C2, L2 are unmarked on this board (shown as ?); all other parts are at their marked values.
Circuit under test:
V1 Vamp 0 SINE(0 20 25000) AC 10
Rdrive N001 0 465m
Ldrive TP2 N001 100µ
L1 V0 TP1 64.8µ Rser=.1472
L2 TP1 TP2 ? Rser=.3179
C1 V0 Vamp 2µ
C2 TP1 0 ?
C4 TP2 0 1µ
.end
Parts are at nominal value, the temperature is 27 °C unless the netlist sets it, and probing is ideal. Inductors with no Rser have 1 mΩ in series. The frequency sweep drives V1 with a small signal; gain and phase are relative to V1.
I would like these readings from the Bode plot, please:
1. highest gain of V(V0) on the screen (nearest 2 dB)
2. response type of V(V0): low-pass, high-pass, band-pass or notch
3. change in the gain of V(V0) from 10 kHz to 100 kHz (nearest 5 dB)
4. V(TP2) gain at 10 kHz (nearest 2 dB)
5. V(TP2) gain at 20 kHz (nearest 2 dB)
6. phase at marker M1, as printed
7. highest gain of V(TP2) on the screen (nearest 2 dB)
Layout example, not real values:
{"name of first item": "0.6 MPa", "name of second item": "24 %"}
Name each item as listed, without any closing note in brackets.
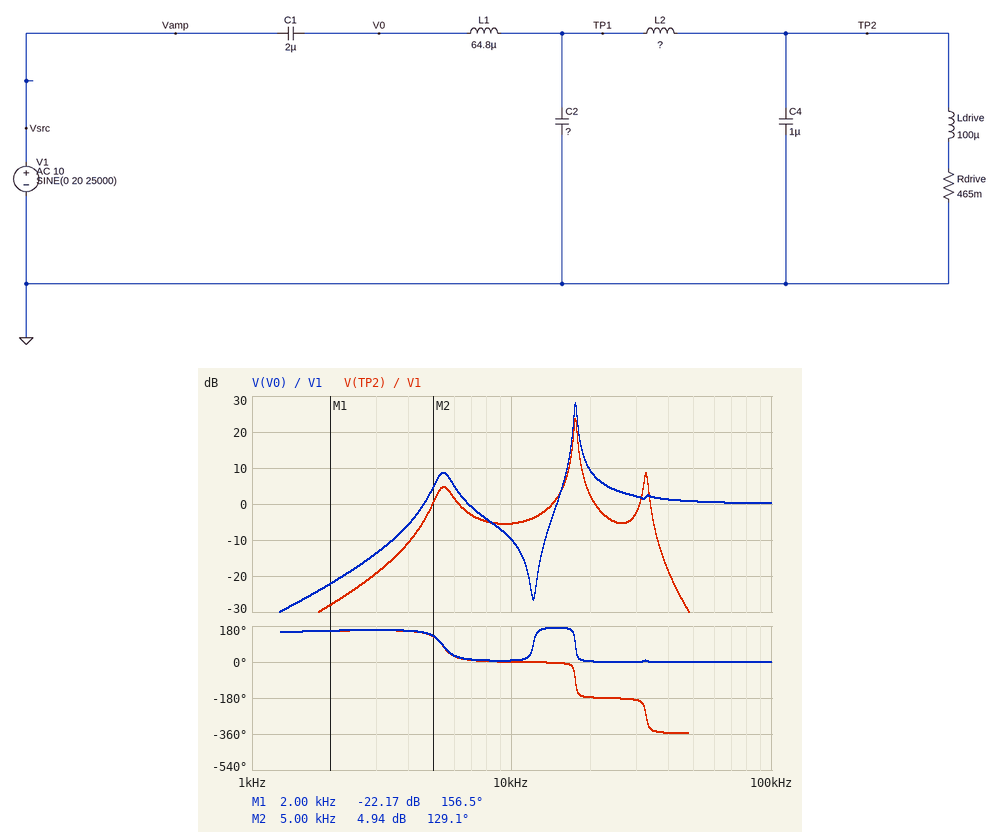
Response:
{"highest gain of V(V0) on the screen": "28 dB", "response type of V(V0): low-pass, high-pass, band-pass or notch": "high-pass", "change in the gain of V(V0) from 10 kHz to 100 kHz": "10 dB", "V(TP2) gain at 10 kHz": "-6 dB", "V(TP2) gain at 20 kHz": "2 dB", "phase at marker M1, as printed": "156.5 deg", "highest gain of V(TP2) on the screen": "24 dB"}
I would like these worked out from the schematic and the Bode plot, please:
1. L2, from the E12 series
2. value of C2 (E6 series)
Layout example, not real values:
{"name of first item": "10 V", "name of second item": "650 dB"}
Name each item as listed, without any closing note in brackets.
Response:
{"L2, from the E12 series": "39 µH", "value of C2": "3.3 µF"}
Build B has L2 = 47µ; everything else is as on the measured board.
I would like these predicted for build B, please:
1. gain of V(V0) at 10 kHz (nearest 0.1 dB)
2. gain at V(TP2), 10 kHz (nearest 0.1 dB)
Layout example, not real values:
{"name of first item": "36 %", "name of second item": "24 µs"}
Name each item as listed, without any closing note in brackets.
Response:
{"gain of V(V0) at 10 kHz": "-10.3 dB", "gain at V(TP2), 10 kHz": "-5.8 dB"}
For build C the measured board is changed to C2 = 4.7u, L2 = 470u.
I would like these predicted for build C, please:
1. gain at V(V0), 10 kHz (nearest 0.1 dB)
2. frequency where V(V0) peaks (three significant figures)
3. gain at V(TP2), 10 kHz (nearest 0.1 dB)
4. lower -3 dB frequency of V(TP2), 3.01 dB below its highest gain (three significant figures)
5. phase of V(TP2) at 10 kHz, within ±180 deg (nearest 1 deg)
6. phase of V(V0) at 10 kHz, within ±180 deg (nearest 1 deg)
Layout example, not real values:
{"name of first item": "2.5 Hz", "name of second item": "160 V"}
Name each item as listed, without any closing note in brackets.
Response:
{"gain at V(V0), 10 kHz": "-25.5 dB", "frequency where V(V0) peaks": "16.6 kHz", "gain at V(TP2), 10 kHz": "-17.9 dB", "lower -3 dB frequency of V(TP2), 3.01 dB below its highest gain": "16.5 kHz", "phase of V(TP2) at 10 kHz, within ±180 deg": "-6 deg", "phase of V(V0) at 10 kHz, within ±180 deg": "155 deg"}
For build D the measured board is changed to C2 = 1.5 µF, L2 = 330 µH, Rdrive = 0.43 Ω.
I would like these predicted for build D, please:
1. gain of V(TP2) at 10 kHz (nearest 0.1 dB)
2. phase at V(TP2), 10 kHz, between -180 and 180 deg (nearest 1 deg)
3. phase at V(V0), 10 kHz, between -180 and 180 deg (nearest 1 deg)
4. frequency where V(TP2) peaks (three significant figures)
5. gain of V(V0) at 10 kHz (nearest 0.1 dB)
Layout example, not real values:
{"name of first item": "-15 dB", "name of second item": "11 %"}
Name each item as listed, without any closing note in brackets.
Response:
{"gain of V(TP2) at 10 kHz": "-11.4 dB", "phase at V(TP2), 10 kHz, between -180 and 180 deg": "-4 deg", "phase at V(V0), 10 kHz, between -180 and 180 deg": "1 deg", "frequency where V(TP2) peaks": "22.4 kHz", "gain of V(V0) at 10 kHz": "-4.4 dB"}
